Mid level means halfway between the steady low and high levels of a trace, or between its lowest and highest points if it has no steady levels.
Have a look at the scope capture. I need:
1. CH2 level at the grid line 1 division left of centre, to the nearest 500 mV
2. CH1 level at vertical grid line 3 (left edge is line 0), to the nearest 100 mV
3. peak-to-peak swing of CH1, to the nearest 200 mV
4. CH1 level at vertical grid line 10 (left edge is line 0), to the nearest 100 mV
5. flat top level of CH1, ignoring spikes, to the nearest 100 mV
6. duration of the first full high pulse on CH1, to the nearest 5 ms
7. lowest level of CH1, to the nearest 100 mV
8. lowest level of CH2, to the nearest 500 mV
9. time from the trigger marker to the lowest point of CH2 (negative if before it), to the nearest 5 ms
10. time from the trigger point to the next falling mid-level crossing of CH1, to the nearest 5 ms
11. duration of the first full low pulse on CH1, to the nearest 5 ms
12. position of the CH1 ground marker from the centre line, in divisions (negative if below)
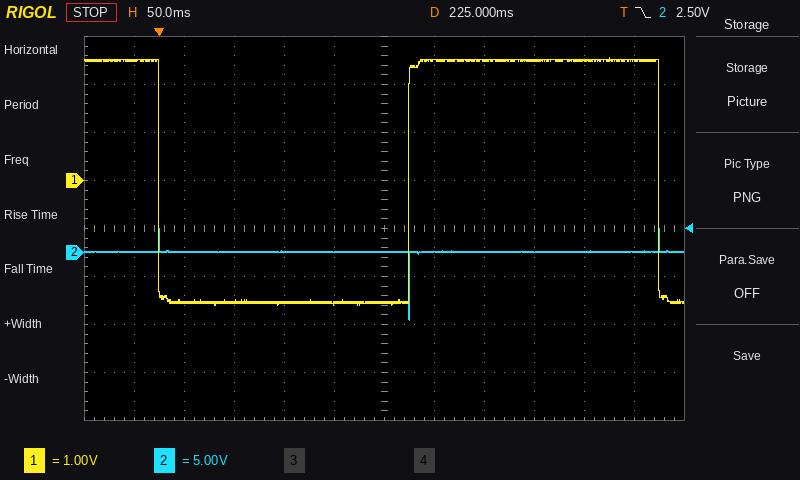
0.0 V
-2.5 V
5.2 V
2.5 V
2.5 V
250 ms
-2.6 V
-7.0 V
+250 ms
500 ms
250 ms
+1.0 div
